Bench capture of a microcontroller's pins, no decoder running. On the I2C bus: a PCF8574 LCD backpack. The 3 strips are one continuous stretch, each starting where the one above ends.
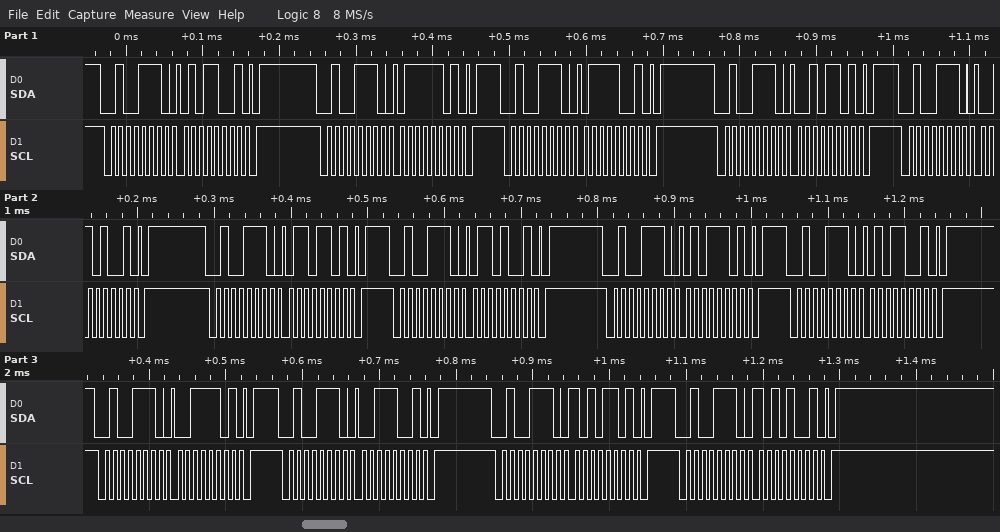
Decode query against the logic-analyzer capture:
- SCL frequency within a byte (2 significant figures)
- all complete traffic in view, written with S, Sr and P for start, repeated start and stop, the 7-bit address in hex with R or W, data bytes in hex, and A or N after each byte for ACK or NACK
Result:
100 kHz
S 27W A 59 A P S 27W A 7D A P S 27W A 79 A P S 27W A 2D A P S 27W A 29 A P S 27W A 6D A P S 27W A 69 A P S 27W A 5D A P S 27W A 59 A P S 27W A 3D A P S 27W A 39 A P S 27W A AD A P S 27W A A9 A P
